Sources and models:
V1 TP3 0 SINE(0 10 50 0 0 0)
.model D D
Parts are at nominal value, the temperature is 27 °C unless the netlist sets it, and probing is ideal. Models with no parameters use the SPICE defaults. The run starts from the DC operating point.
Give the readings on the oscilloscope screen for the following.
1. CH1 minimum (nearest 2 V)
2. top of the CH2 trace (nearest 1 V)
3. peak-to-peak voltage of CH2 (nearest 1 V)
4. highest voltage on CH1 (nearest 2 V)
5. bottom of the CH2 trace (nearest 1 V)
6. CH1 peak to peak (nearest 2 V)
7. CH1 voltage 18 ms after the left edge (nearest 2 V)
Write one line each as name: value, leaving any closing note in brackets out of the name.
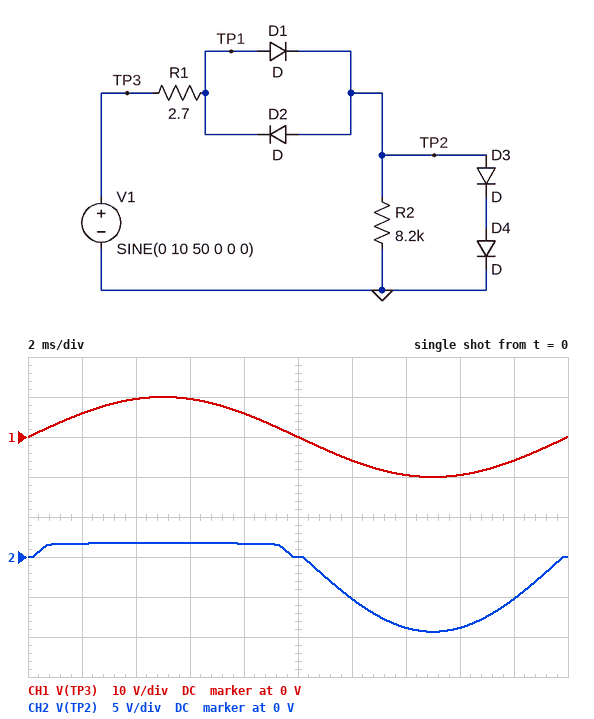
CH1 minimum: -10 V
top of the CH2 trace: 2 V
peak-to-peak voltage of CH2: 11 V
highest voltage on CH1: 10 V
bottom of the CH2 trace: -9 V
CH1 peak to peak: 20 V
CH1 voltage 18 ms after the left edge: -6 V
